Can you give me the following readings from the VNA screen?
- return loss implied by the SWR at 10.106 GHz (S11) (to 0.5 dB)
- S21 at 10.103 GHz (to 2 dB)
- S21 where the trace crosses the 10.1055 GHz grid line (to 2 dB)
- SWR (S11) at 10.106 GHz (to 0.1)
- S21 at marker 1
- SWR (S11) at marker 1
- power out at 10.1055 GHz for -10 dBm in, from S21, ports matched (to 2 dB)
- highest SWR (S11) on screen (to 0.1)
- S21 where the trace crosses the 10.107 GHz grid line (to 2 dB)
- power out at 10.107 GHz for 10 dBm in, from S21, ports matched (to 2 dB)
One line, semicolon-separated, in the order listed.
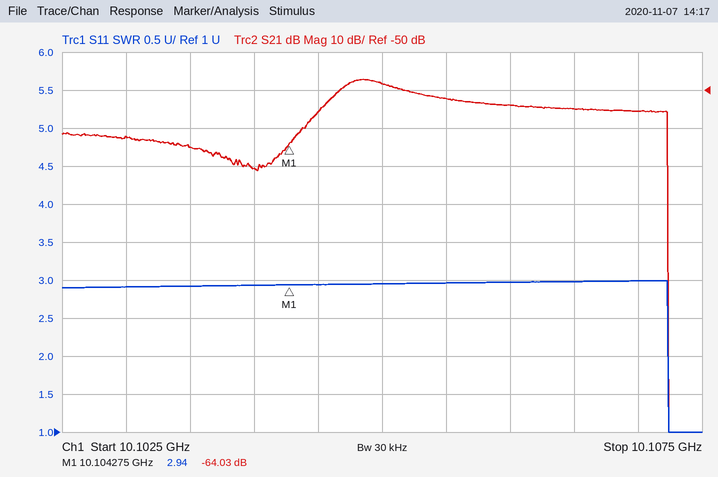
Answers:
6.0 dB; -62 dB; -52 dB; 3.0; -64.03 dB; 2.94; -62 dBm; 3.0; -56 dB; -46 dBm
